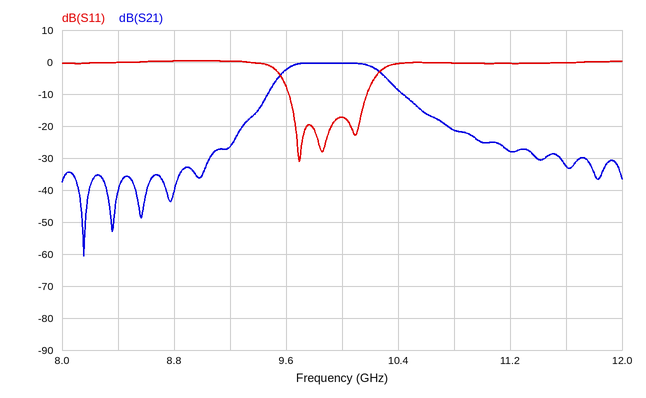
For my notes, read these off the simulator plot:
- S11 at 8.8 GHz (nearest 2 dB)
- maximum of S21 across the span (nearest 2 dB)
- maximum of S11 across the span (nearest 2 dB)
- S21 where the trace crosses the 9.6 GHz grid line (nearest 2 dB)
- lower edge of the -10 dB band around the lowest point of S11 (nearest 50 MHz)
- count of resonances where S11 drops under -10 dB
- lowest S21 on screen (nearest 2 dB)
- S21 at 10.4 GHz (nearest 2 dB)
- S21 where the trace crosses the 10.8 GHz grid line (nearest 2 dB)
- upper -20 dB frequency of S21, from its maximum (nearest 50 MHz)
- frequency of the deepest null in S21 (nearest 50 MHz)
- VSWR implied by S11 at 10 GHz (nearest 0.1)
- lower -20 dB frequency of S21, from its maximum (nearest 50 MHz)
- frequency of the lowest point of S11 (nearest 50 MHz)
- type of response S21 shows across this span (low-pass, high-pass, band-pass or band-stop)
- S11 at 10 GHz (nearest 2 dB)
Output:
0 dB
0 dB
0 dB
-2 dB
9.60 GHz
3
-60 dB
-8 dB
-22 dB
10.75 GHz
8.15 GHz
1.3
9.30 GHz
9.70 GHz
band-pass
-18 dB
